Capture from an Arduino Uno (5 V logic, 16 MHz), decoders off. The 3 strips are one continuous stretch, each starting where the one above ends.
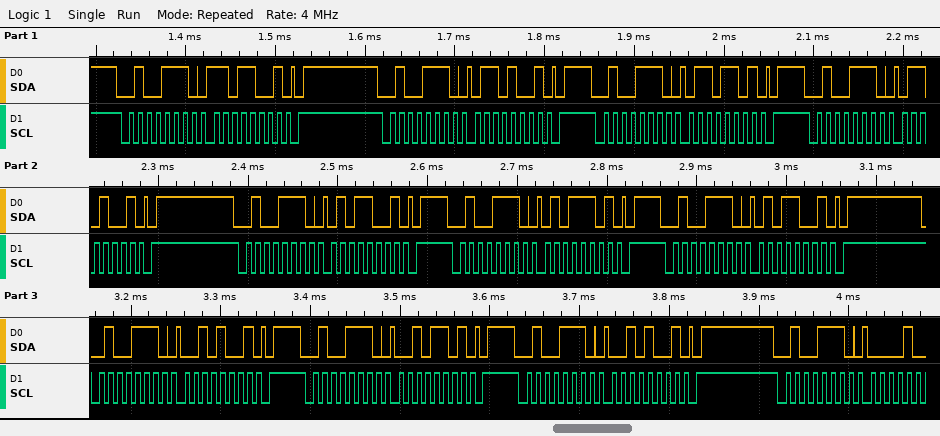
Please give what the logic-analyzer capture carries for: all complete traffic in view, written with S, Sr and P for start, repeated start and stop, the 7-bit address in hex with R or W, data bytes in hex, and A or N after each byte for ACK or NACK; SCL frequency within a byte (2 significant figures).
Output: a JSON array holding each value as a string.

["S 27W A D9 A P S 27W A 69 A P S 27W A 6D A P S 27W A 69 A P S 27W A 59 A P S 27W A 5D A P S 27W A 59 A P S 27W A 29 A P S 27W A 2D A P S 27W A 29 A P S 27W A", "100 kHz"]
